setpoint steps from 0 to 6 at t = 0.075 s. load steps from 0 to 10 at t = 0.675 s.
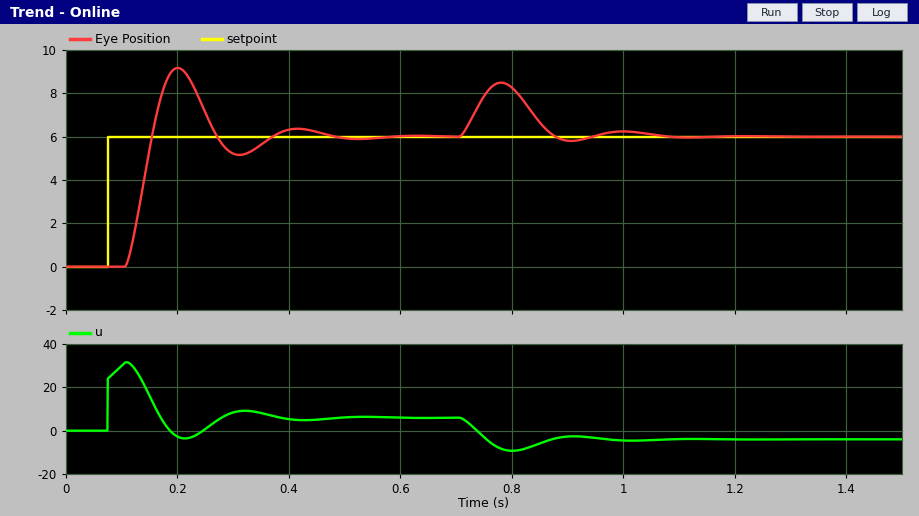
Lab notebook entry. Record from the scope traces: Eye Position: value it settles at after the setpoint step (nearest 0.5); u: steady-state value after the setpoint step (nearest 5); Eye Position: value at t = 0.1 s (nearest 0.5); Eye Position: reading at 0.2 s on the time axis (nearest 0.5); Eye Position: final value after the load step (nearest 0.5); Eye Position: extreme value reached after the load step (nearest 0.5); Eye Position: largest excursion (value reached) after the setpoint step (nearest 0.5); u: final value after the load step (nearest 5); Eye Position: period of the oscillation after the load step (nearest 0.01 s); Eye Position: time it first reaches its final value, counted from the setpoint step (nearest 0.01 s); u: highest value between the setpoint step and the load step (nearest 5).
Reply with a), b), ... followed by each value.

a) 6.0
b) 5
c) 0.0
d) 9.0
e) 6.0
f) 8.5
g) 9.0
h) -5
i) 0.22 s
j) 0.08 s
k) 30
